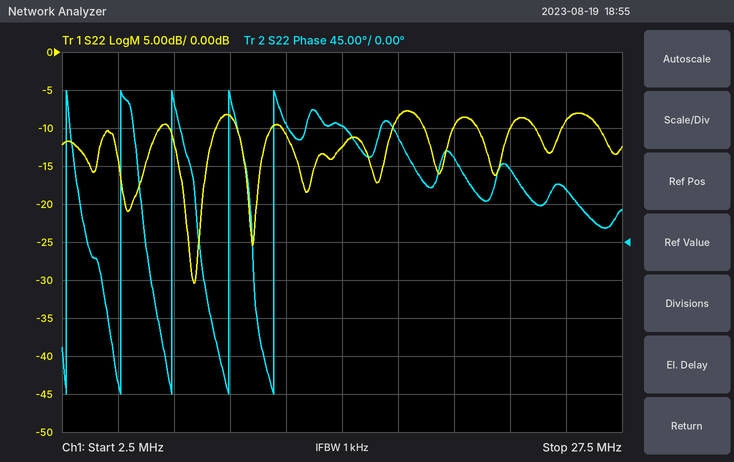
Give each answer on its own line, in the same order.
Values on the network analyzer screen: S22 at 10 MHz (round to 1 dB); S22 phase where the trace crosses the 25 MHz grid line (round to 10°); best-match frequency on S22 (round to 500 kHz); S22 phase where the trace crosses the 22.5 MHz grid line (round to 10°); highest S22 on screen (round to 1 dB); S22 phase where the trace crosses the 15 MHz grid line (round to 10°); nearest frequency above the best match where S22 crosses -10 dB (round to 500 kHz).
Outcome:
-8 dB
60°
8.5 MHz
90°
-8 dB
140°
9.5 MHz
